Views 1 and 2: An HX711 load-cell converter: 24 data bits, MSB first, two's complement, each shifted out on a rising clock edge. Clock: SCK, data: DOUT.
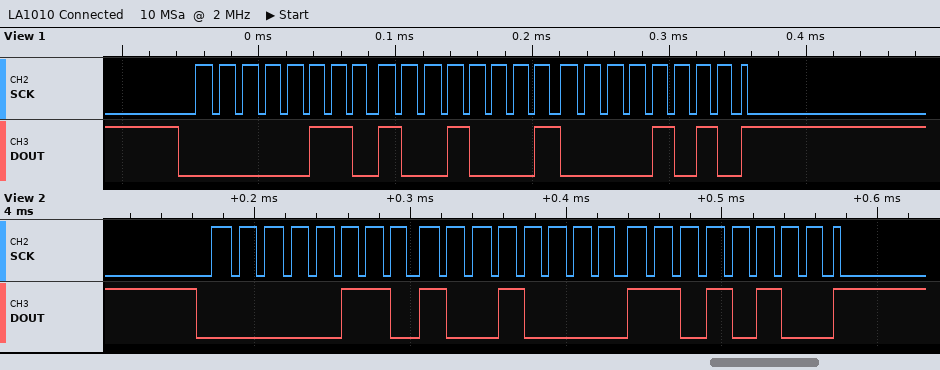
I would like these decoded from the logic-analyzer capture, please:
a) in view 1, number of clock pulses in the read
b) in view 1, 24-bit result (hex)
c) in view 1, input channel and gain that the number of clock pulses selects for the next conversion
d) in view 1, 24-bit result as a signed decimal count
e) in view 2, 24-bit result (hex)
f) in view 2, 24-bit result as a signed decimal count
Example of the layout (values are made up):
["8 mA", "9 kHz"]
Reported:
["25", "0x06910A", "channel A, gain 128", "430346", "0x0690D4", "430292"]
